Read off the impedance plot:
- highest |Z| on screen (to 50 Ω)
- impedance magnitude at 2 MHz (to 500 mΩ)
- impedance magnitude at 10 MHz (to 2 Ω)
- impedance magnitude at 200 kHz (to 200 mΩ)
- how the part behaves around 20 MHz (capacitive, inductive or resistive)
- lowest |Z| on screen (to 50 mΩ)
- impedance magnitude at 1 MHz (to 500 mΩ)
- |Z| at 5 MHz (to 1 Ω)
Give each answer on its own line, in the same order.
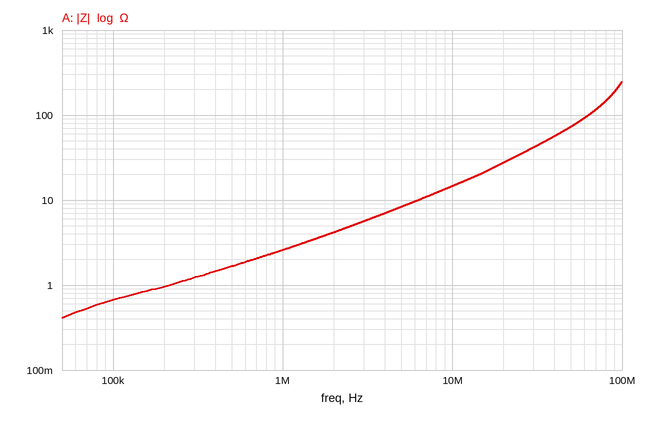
250 Ω
4.0 Ω
14 Ω
1.0 Ω
inductive
400 mΩ
2.5 Ω
8 Ω
